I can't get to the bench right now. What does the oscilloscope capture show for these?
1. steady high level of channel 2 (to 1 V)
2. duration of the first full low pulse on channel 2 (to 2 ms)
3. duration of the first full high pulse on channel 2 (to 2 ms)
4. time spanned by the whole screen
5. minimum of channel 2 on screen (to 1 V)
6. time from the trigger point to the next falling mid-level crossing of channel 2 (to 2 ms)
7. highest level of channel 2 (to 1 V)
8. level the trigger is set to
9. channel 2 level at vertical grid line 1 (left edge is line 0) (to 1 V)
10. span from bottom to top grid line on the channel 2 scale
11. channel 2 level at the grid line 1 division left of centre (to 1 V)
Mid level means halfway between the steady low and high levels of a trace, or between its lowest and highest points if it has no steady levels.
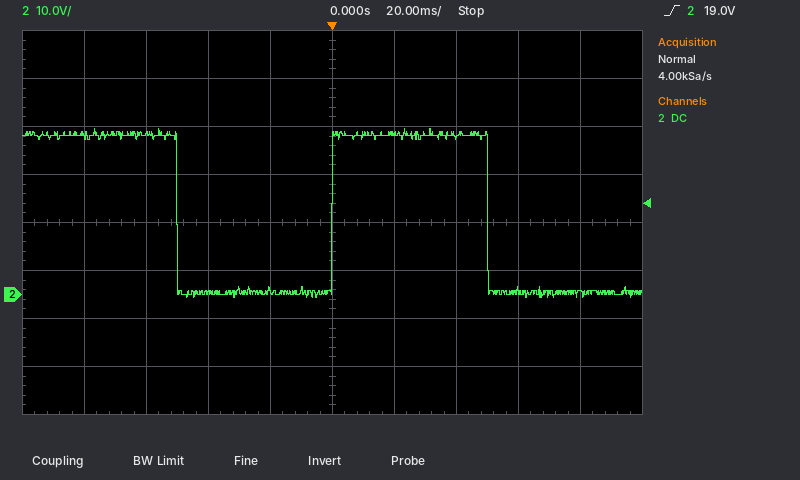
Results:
33 V
50 ms
50 ms
200 ms
-1 V
50 ms
35 V
19.0 V
33 V
80 V
1 V
